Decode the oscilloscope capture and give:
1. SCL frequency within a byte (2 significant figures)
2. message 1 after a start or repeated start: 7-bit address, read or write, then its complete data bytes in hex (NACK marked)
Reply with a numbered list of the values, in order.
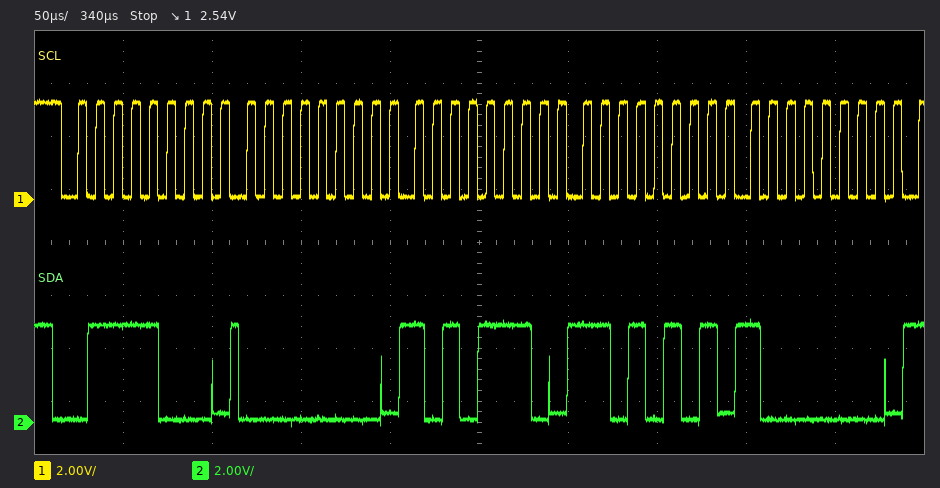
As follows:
1. 100 kHz
2. 0x3C write: 00 AE D5 80
